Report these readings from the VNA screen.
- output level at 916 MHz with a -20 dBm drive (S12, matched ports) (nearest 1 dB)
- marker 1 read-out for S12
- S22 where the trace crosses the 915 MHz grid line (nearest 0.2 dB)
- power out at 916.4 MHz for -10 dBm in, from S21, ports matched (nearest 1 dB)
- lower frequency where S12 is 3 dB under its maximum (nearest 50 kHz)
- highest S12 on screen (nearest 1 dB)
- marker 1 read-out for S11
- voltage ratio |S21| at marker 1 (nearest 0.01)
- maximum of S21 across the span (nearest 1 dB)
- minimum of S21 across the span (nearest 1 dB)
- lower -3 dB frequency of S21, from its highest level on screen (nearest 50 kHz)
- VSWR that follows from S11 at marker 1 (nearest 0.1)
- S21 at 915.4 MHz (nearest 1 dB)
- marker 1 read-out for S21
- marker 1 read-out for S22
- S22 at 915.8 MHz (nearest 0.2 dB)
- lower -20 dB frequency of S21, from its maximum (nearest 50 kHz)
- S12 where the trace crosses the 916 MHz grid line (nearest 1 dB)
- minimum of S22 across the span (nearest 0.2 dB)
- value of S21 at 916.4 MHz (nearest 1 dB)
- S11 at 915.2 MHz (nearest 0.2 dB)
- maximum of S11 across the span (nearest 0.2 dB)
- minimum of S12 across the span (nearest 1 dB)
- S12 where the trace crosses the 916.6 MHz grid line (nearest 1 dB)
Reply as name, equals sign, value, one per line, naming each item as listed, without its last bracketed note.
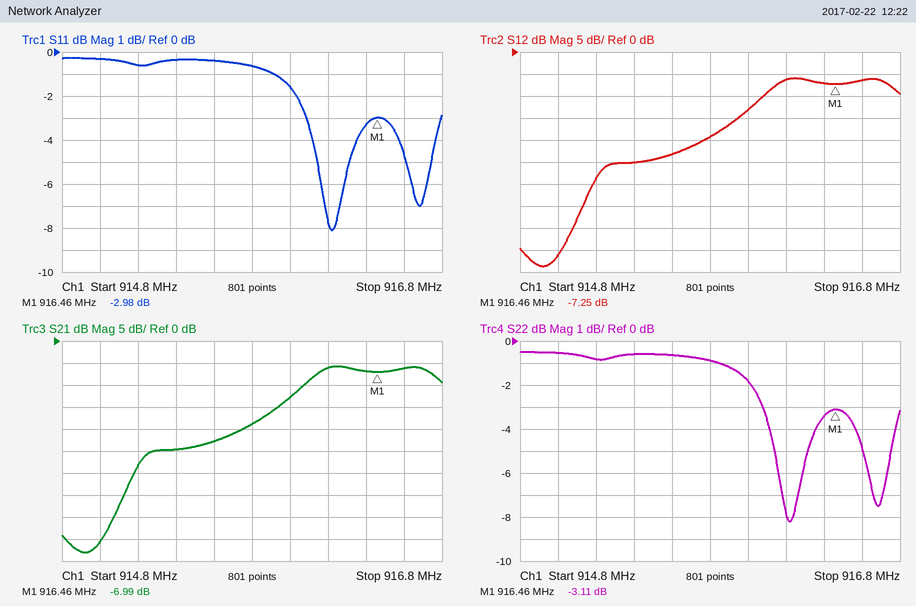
output level at 916 MHz with a -20 dBm drive (S12, matched ports) = -33 dBm
marker 1 read-out for S12 = -7.25 dB
S22 where the trace crosses the 915 MHz grid line = -0.6 dB
power out at 916.4 MHz for -10 dBm in, from S21, ports matched = -17 dBm
lower frequency where S12 is 3 dB under its maximum = 916.10 MHz
highest S12 on screen = -6 dB
marker 1 read-out for S11 = -2.98 dB
voltage ratio |S21| at marker 1 = 0.45
maximum of S21 across the span = -6 dB
minimum of S21 across the span = -48 dB
lower -3 dB frequency of S21, from its highest level on screen = 916.10 MHz
VSWR that follows from S11 at marker 1 = 5.9
S21 at 915.4 MHz = -25 dB
marker 1 read-out for S21 = -6.99 dB
marker 1 read-out for S22 = -3.11 dB
S22 at 915.8 MHz = -0.8 dB
lower -20 dB frequency of S21, from its maximum = 915.25 MHz
S12 where the trace crosses the 916 MHz grid line = -13 dB
minimum of S22 across the span = -8.2 dB
value of S21 at 916.4 MHz = -7 dB
S11 at 915.2 MHz = -0.6 dB
maximum of S11 across the span = -0.2 dB
minimum of S12 across the span = -49 dB
S12 where the trace crosses the 916.6 MHz grid line = -6 dB
